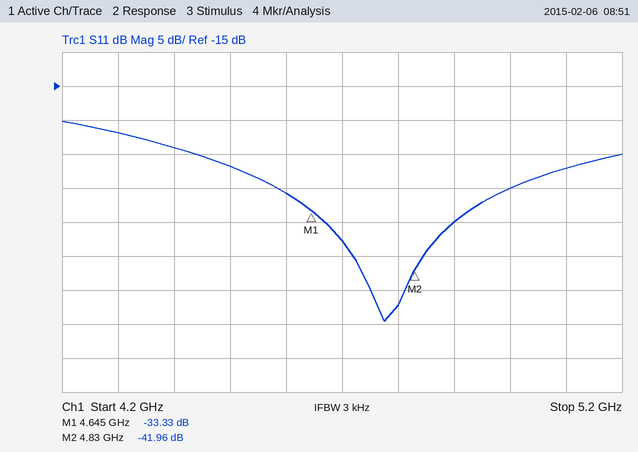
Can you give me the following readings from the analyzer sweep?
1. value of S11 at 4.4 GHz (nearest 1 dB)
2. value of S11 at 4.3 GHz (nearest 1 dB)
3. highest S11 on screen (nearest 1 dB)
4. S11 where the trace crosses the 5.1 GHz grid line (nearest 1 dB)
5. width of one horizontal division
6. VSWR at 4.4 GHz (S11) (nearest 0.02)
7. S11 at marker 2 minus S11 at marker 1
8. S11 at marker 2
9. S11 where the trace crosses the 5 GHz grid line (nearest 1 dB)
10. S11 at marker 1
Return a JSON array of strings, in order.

["-24 dB", "-22 dB", "-20 dB", "-27 dB", "100 MHz", "1.14", "-8.63 dB", "-41.96 dB", "-30 dB", "-33.33 dB"]
